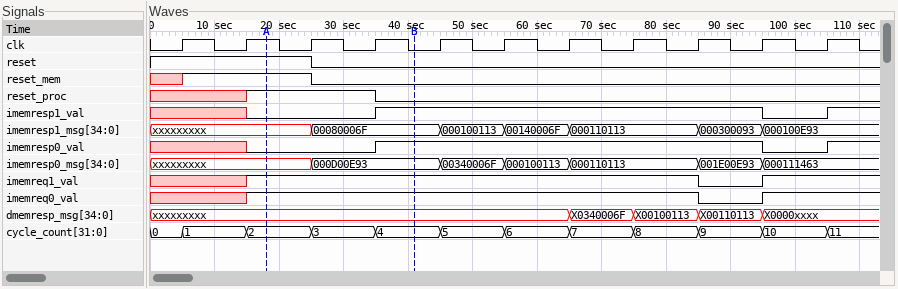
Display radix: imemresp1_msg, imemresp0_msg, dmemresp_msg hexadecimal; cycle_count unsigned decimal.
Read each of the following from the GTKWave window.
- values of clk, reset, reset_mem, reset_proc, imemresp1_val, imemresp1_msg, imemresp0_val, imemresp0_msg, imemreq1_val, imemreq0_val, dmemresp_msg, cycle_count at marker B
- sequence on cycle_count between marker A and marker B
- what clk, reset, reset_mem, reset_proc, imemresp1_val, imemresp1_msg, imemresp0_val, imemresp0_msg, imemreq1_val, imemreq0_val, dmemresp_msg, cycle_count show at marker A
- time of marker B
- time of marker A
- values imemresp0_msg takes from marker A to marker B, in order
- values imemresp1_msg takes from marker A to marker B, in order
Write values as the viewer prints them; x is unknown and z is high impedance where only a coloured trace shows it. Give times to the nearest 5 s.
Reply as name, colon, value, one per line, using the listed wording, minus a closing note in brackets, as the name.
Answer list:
values of clk, reset, reset_mem, reset_proc, imemresp1_val, imemresp1_msg, imemresp0_val, imemresp0_msg, imemreq1_val, imemreq0_val, dmemresp_msg, cycle_count at marker B: clk=0, reset=0, reset_mem=0, reset_proc=0, imemresp1_val=1, imemresp1_msg=00080006F, imemresp0_val=1, imemresp0_msg=000D00E93, imemreq1_val=1, imemreq0_val=1, dmemresp_msg=xxxxxxxxx, cycle_count=4
sequence on cycle_count between marker A and marker B: 2, 3, 4
what clk, reset, reset_mem, reset_proc, imemresp1_val, imemresp1_msg, imemresp0_val, imemresp0_msg, imemreq1_val, imemreq0_val, dmemresp_msg, cycle_count show at marker A: clk=1, reset=1, reset_mem=1, reset_proc=1, imemresp1_val=0, imemresp1_msg=xxxxxxxxx, imemresp0_val=0, imemresp0_msg=xxxxxxxxx, imemreq1_val=1, imemreq0_val=1, dmemresp_msg=xxxxxxxxx, cycle_count=2
time of marker B: 40 s
time of marker A: 20 s
values imemresp0_msg takes from marker A to marker B, in order: xxxxxxxxx, 000D00E93
values imemresp1_msg takes from marker A to marker B, in order: xxxxxxxxx, 00080006F
